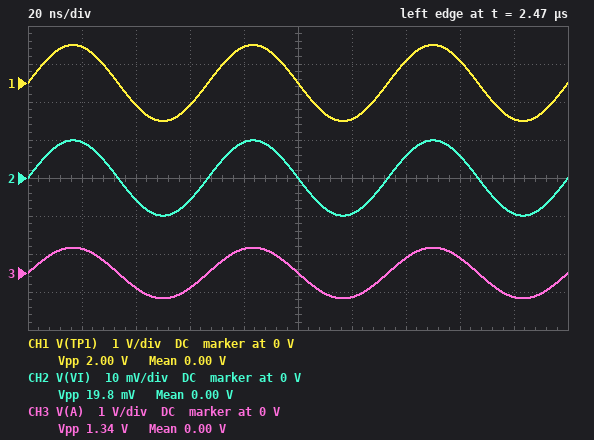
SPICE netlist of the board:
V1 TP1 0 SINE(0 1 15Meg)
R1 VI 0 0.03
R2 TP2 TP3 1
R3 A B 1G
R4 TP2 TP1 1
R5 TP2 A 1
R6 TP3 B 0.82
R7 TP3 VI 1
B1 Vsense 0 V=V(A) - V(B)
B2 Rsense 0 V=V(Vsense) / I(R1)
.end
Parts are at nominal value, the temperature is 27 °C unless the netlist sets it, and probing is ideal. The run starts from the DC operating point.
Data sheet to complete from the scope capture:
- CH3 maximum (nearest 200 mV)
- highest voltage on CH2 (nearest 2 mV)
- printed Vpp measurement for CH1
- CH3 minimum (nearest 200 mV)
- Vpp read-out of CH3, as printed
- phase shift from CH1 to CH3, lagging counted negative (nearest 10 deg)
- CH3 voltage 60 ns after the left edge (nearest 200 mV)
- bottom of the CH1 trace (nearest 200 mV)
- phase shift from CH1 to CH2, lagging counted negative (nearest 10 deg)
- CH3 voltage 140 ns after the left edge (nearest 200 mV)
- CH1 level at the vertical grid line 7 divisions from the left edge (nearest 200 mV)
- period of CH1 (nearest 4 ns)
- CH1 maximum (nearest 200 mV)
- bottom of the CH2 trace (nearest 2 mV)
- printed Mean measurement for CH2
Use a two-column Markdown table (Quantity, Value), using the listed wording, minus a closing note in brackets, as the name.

| Quantity | Value |
|---|---|
| CH3 maximum | 600 mV |
| highest voltage on CH2 | 10 mV |
| printed Vpp measurement for CH1 | 2.00 V |
| CH3 minimum | -600 mV |
| Vpp read-out of CH3, as printed | 1.34 V |
| phase shift from CH1 to CH3, lagging counted negative | 0 deg |
| CH3 voltage 60 ns after the left edge | -400 mV |
| bottom of the CH1 trace | -1.0 V |
| phase shift from CH1 to CH2, lagging counted negative | 0 deg |
| CH3 voltage 140 ns after the left edge | 400 mV |
| CH1 level at the vertical grid line 7 divisions from the left edge | 600 mV |
| period of CH1 | 68 ns |
| CH1 maximum | 1.0 V |
| bottom of the CH2 trace | -10 mV |
| printed Mean measurement for CH2 | 0.00 V |
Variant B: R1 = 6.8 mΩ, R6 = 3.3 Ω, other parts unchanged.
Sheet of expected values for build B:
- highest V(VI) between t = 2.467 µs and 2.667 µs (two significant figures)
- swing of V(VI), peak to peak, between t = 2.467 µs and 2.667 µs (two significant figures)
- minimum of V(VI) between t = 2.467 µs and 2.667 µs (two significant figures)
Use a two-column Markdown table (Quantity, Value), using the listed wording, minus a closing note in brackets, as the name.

| Quantity | Value |
|---|---|
| highest V(VI) between t = 2.467 µs and 2.667 µs | 2.3 mV |
| swing of V(VI), peak to peak, between t = 2.467 µs and 2.667 µs | 4.5 mV |
| minimum of V(VI) between t = 2.467 µs and 2.667 µs | -2.3 mV |
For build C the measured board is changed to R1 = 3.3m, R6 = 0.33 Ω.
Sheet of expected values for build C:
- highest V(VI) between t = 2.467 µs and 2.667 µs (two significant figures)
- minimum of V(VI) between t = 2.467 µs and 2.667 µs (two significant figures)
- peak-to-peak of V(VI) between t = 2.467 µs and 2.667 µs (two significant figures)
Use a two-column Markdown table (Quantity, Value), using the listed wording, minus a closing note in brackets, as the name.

| Quantity | Value |
|---|---|
| highest V(VI) between t = 2.467 µs and 2.667 µs | 1.1 mV |
| minimum of V(VI) between t = 2.467 µs and 2.667 µs | -1.1 mV |
| peak-to-peak of V(VI) between t = 2.467 µs and 2.667 µs | 2.2 mV |
